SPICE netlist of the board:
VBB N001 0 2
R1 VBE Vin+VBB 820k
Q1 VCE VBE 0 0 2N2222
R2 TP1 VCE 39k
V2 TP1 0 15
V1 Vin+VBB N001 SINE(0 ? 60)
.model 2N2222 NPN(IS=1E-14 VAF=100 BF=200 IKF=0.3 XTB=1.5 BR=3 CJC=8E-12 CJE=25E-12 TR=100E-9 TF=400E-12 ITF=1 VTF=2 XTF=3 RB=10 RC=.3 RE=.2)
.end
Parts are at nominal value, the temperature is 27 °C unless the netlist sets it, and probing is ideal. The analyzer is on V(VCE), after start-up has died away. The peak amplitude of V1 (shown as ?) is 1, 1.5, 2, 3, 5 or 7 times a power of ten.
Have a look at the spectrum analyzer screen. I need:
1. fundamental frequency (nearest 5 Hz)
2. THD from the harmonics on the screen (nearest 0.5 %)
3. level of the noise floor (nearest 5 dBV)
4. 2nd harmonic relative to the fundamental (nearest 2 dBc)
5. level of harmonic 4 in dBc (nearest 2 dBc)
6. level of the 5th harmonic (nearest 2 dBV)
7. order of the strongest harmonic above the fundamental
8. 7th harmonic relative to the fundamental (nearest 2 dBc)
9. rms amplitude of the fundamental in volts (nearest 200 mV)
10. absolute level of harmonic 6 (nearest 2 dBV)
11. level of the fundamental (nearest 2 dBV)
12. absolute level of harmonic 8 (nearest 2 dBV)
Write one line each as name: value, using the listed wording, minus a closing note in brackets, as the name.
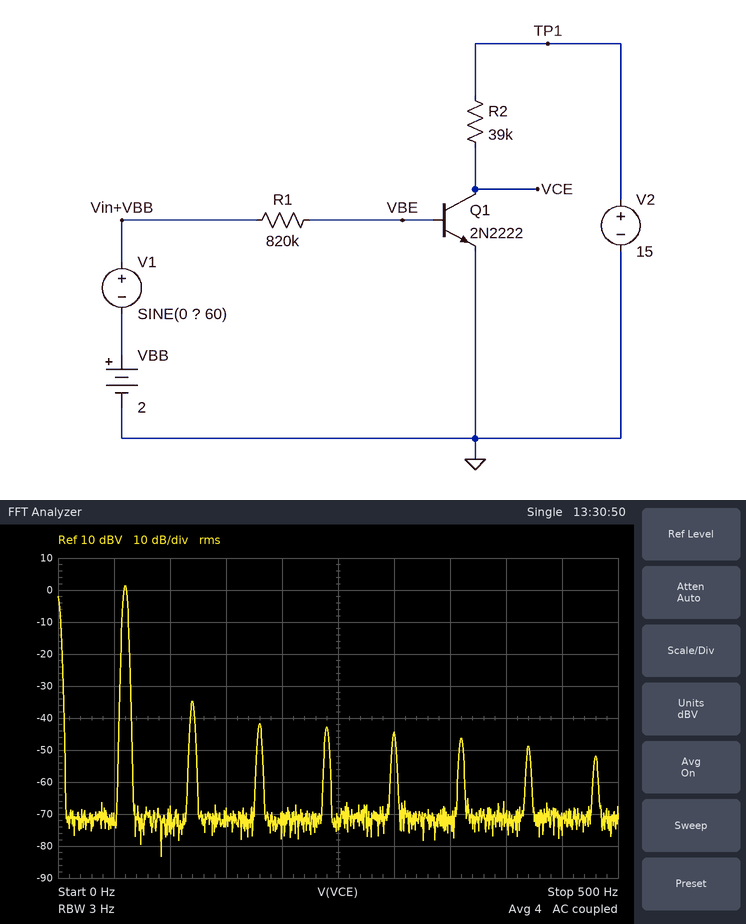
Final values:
fundamental frequency: 60 Hz
THD from the harmonics on the screen: 2.0 %
level of the noise floor: -70 dBV
2nd harmonic relative to the fundamental: -36 dBc
level of harmonic 4 in dBc: -44 dBc
level of the 5th harmonic: -44 dBV
order of the strongest harmonic above the fundamental: 2
7th harmonic relative to the fundamental: -50 dBc
rms amplitude of the fundamental in volts: 1.2 V
absolute level of harmonic 6: -46 dBV
level of the fundamental: 2 dBV
absolute level of harmonic 8: -52 dBV
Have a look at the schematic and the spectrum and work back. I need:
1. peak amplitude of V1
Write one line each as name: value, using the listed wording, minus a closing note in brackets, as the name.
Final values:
peak amplitude of V1: 200 mV
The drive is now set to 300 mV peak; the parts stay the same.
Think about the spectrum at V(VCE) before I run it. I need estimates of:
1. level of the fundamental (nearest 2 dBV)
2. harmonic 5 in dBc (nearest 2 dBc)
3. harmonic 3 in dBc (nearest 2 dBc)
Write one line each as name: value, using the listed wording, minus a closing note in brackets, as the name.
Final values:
level of the fundamental: 4 dBV
harmonic 5 in dBc: -50 dBc
harmonic 3 in dBc: -24 dBc
